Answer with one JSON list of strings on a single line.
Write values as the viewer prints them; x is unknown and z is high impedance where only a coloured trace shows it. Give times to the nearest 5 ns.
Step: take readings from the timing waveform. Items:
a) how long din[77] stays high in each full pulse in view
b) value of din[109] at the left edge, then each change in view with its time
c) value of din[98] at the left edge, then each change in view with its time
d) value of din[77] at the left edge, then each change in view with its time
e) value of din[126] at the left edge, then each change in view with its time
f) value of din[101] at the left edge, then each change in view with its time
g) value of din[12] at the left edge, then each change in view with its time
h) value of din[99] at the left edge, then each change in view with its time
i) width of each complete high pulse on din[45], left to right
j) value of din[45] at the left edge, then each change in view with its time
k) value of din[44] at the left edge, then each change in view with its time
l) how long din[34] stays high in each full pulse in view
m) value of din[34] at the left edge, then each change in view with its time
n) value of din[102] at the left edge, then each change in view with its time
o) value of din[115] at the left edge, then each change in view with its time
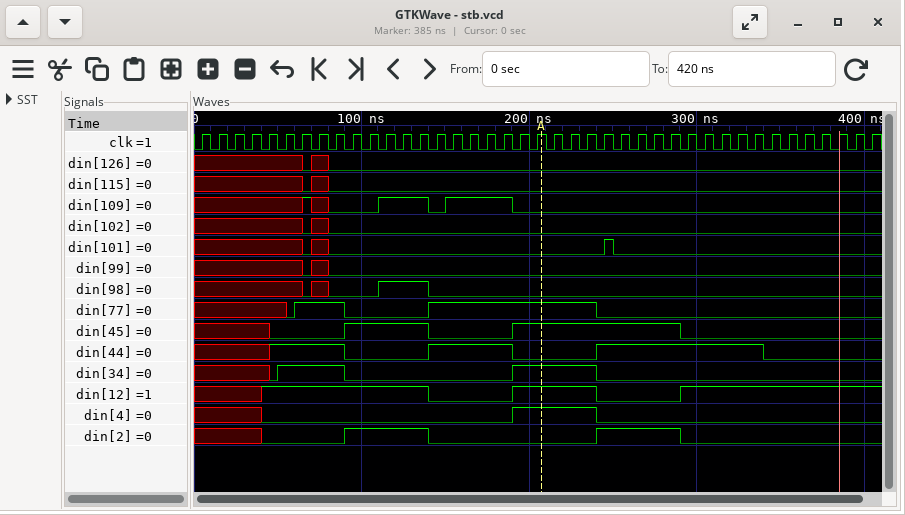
["30 ns, 100 ns", "x, 1 at 65 ns, x at 70 ns, 0 at 80 ns, 1 at 110 ns, 0 at 140 ns, 1 at 150 ns, 0 at 190 ns", "x, 0 at 65 ns, x at 70 ns, 0 at 80 ns, 1 at 110 ns, 0 at 140 ns", "x, 0 at 55 ns, 1 at 60 ns, 0 at 90 ns, 1 at 140 ns, 0 at 240 ns", "x, 0 at 65 ns, x at 70 ns, 0 at 80 ns", "x, 0 at 65 ns, x at 70 ns, 0 at 80 ns, 1 at 245 ns, 0 at 250 ns", "x, 1 at 40 ns, 0 at 140 ns, 1 at 190 ns, 0 at 240 ns, 1 at 290 ns", "x, 0 at 65 ns, x at 70 ns, 0 at 80 ns", "50 ns, 100 ns", "x, 0 at 45 ns, 1 at 90 ns, 0 at 140 ns, 1 at 190 ns, 0 at 290 ns", "x, 1 at 45 ns, 0 at 90 ns, 1 at 140 ns, 0 at 190 ns, 1 at 240 ns, 0 at 340 ns", "40 ns, 50 ns", "x, 0 at 45 ns, 1 at 50 ns, 0 at 90 ns, 1 at 190 ns, 0 at 240 ns", "x, 0 at 65 ns, x at 70 ns, 0 at 80 ns", "x, 0 at 65 ns, x at 70 ns, 0 at 80 ns"]
